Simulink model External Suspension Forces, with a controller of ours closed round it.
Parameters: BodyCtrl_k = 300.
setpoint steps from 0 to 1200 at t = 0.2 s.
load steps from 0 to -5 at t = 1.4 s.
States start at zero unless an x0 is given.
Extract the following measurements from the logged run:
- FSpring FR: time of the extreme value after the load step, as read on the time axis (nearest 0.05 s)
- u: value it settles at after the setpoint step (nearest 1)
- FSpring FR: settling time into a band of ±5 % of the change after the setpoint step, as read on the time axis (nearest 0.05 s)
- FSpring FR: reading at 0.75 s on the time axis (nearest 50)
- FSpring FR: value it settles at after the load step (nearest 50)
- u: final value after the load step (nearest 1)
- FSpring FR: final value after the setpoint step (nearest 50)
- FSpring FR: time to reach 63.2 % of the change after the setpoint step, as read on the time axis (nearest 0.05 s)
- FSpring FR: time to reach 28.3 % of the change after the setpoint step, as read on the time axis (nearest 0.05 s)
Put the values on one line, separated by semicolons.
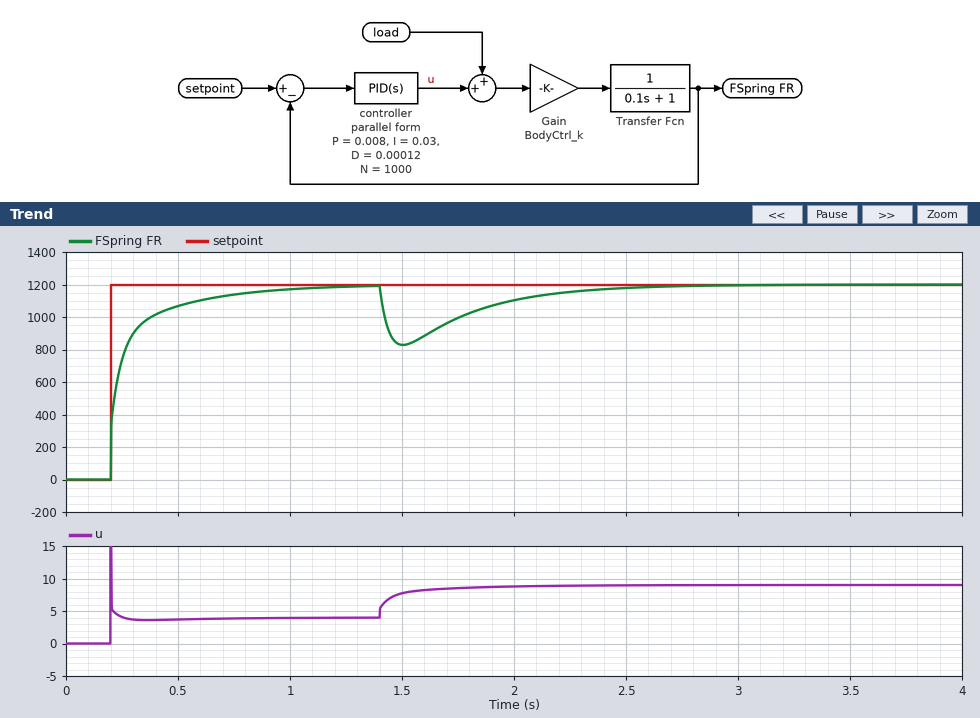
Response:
1.50 s; 4; 0.75 s; 1150; 1200; 9; 1200; 0.25 s; 0.20 s
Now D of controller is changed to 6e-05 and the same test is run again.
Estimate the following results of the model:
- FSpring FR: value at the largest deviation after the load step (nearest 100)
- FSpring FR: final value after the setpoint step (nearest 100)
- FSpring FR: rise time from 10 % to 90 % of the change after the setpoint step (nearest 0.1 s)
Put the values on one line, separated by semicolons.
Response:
800; 1200; 0.3 s
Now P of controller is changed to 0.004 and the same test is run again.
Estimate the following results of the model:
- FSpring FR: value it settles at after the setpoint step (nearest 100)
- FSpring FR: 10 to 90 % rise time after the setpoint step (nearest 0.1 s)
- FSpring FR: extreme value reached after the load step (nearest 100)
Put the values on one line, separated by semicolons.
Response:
1200; 0.3 s; 700
